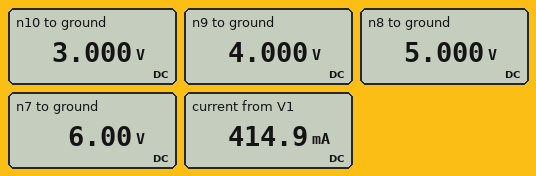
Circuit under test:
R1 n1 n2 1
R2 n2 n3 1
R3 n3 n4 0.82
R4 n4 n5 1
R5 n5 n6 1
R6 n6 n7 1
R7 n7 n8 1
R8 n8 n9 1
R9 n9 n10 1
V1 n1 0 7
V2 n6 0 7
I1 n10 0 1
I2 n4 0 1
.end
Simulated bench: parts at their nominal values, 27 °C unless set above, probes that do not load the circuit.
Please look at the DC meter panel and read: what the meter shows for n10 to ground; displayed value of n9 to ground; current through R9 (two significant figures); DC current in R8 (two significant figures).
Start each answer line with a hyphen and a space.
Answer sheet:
- 3.000 V
- 4.000 V
- 1.0 A
- 1.0 A
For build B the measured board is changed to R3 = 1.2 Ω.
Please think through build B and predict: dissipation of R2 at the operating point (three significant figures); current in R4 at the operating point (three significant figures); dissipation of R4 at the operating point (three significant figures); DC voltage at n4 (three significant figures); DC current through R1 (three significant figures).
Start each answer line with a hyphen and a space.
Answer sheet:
- 148 mW
- 615 mA
- 379 mW
- 5.77 V
- 385 mA
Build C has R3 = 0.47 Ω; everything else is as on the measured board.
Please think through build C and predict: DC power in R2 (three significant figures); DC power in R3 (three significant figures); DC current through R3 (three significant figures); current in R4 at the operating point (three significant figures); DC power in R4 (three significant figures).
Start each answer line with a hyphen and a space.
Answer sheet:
- 200 mW
- 94.1 mW
- 447 mA
- 553 mA
- 305 mW
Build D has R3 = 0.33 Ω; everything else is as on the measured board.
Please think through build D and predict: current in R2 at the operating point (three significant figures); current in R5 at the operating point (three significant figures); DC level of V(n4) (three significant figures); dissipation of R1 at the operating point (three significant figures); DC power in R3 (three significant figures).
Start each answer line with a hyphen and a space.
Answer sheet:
- 462 mA
- 538 mA
- 5.92 V
- 213 mW
- 70.4 mW
